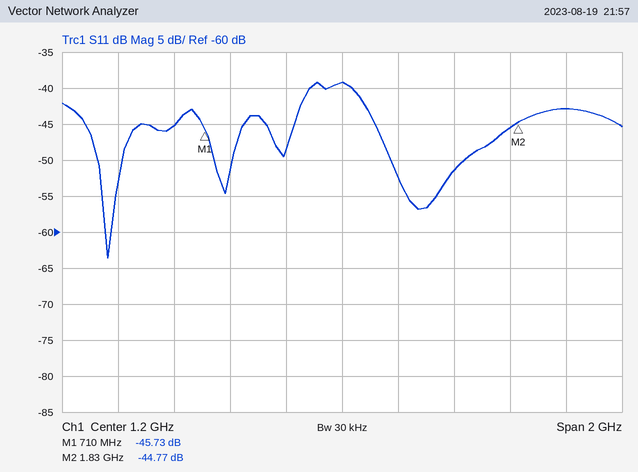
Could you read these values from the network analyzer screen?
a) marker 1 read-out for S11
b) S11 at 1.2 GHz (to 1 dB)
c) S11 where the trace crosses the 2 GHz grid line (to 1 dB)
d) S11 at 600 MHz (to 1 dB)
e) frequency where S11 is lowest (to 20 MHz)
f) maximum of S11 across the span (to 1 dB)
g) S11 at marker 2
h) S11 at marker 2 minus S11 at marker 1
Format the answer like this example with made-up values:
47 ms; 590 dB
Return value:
-45.73 dB; -39 dB; -43 dB; -45 dB; 360 MHz; -39 dB; -44.77 dB; 0.96 dB
